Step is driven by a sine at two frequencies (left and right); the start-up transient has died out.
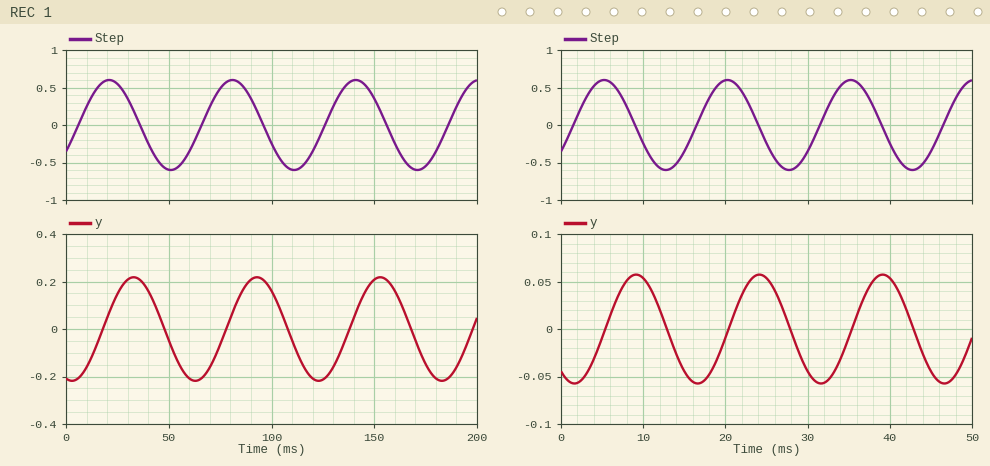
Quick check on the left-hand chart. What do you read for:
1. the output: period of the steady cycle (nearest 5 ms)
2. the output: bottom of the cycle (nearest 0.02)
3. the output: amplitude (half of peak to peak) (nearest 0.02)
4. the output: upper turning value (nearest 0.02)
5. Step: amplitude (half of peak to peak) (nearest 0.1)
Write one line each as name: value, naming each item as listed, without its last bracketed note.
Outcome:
the output: period of the steady cycle: 60 ms
the output: bottom of the cycle: -0.22
the output: amplitude (half of peak to peak): 0.22
the output: upper turning value: 0.22
Step: amplitude (half of peak to peak): 0.6
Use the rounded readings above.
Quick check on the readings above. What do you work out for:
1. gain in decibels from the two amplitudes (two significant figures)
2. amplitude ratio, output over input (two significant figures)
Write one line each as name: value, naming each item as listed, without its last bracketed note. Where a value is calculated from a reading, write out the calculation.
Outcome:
gain in decibels from the two amplitudes: 20 log10(0.22 / 0.6) = -8.7 dB
amplitude ratio, output over input: 0.22 / 0.6 = 0.37
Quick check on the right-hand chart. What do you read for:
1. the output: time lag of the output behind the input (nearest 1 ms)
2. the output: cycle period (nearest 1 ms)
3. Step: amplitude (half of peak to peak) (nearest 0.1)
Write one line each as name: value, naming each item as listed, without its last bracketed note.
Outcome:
the output: time lag of the output behind the input: 4 ms
the output: cycle period: 15 ms
Step: amplitude (half of peak to peak): 0.6
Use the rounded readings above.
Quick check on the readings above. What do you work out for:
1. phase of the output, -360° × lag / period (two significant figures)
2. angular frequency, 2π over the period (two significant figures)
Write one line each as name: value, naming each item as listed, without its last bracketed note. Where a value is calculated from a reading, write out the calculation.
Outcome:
phase of the output, -360° × lag / period: -360 × 4 / 15 = -96°
angular frequency, 2π over the period: 2π / 15 = 0.42 rad/ms
